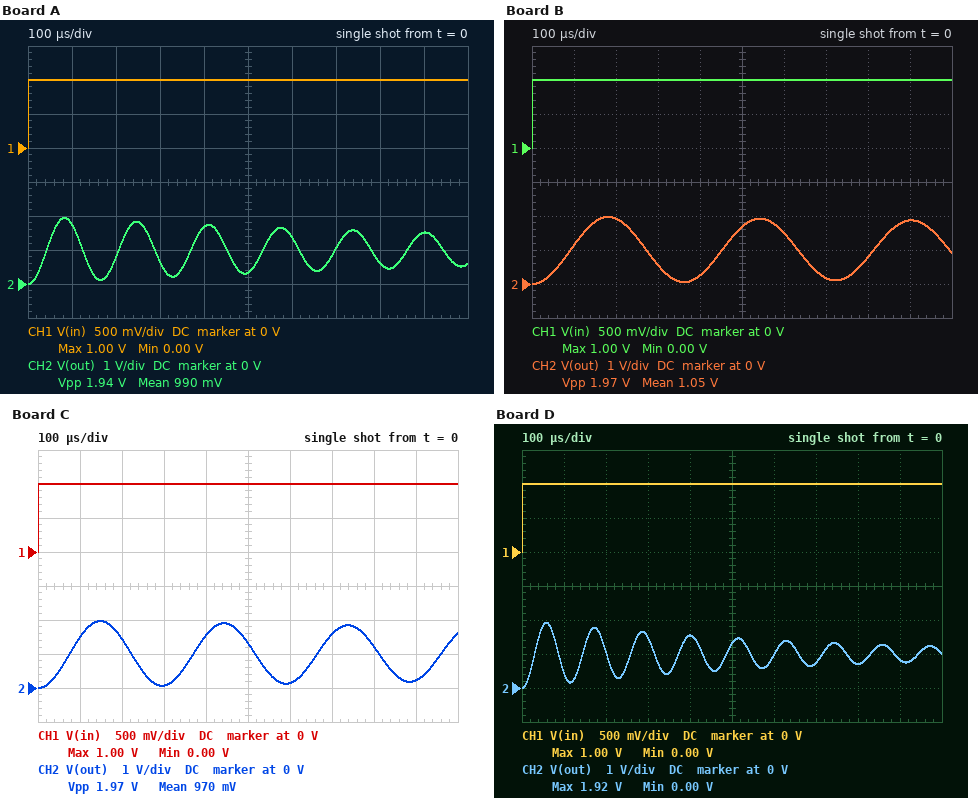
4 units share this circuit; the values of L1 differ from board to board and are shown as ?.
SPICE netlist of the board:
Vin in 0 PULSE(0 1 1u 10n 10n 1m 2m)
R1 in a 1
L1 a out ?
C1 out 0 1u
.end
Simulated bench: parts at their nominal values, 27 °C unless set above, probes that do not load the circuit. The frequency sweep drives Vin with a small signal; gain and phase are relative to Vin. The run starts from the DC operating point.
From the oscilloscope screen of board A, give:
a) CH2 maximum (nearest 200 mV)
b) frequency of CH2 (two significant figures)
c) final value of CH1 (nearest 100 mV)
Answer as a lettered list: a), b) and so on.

a) 2.0 V
b) 6.1 kHz
c) 1.0 V
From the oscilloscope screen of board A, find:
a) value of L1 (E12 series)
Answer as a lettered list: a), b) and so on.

a) 680 µH
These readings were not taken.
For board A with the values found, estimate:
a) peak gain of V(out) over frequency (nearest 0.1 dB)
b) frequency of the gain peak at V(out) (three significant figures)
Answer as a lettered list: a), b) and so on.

a) 28.3 dB
b) 6.10 kHz
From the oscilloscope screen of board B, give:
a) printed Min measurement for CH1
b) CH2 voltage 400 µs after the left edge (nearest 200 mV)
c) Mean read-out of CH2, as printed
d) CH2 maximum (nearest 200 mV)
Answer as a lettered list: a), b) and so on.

a) 0.00 V
b) 200 mV
c) 1.05 V
d) 2.0 V
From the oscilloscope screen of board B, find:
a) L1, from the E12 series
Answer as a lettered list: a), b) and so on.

a) 3.3 mH
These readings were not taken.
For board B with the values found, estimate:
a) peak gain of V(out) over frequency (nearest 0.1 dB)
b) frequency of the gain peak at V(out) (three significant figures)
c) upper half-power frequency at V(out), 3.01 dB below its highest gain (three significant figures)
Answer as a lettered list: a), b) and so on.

a) 35.2 dB
b) 2.77 kHz
c) 2.79 kHz
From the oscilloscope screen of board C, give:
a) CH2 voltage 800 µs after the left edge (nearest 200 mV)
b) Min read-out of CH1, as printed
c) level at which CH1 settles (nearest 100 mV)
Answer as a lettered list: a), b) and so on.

a) 1.2 V
b) 0.00 V
c) 1.0 V
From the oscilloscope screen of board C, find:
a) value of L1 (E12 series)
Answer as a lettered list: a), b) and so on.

a) 2.2 mH
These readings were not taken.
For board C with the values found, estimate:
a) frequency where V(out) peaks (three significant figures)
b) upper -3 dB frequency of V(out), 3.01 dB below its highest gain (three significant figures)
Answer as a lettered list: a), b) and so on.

a) 3.39 kHz
b) 3.43 kHz
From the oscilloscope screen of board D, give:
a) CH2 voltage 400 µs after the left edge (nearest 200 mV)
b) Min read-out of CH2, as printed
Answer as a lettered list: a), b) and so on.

a) 1.6 V
b) 0.00 V
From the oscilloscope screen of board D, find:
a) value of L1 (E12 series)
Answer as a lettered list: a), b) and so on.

a) 330 µH
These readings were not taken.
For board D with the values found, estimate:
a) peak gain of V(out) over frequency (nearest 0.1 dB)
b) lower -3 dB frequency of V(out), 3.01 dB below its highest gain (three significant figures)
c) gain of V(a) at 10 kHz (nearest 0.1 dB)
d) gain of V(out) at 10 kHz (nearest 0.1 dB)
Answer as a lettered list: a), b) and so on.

a) 25.2 dB
b) 8.51 kHz
c) -0.2 dB
d) 10.2 dB
